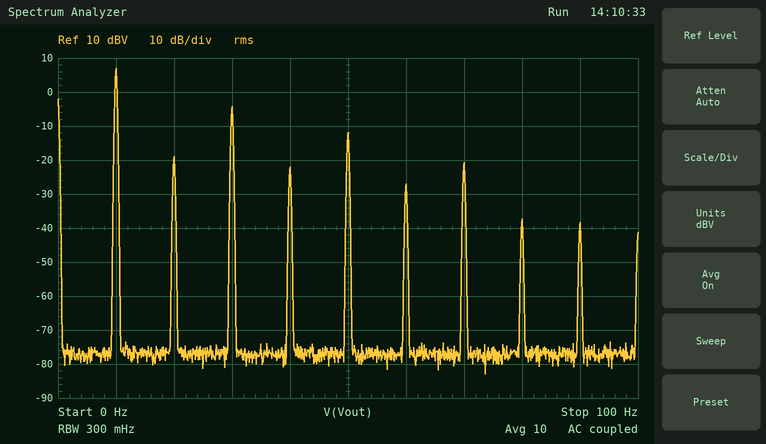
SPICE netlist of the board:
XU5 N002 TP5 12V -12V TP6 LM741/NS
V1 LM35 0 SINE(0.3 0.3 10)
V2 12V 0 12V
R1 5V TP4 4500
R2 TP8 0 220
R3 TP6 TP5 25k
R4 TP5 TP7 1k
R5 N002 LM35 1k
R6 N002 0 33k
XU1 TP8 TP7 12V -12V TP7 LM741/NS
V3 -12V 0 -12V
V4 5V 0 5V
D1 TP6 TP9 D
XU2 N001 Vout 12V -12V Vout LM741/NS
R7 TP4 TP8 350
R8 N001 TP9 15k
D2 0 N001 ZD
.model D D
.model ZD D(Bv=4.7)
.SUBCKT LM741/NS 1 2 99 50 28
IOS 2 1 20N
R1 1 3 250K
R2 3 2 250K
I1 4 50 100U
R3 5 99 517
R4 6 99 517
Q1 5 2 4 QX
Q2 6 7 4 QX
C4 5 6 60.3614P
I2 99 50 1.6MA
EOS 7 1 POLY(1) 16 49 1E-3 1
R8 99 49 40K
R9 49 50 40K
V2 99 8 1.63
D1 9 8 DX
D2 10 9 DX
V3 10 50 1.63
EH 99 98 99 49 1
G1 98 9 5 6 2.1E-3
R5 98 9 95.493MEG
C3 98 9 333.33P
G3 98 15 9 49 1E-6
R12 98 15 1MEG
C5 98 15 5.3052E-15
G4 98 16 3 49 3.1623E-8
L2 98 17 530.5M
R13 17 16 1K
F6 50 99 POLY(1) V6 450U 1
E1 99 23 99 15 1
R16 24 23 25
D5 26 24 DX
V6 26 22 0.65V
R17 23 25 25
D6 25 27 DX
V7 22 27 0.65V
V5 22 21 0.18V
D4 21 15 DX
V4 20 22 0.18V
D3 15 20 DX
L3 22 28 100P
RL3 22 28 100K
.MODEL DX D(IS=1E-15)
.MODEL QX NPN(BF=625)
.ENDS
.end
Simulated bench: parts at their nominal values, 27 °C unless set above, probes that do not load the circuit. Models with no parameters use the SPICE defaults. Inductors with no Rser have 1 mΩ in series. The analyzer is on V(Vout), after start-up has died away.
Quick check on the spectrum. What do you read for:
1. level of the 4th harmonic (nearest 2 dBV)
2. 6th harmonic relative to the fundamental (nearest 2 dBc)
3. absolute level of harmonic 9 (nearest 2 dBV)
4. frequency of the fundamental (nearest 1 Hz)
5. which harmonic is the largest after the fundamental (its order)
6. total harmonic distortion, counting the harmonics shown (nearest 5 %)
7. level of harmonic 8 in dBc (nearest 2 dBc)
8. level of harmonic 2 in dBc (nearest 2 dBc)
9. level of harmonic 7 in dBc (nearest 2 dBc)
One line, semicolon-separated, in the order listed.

-22 dBV; -34 dBc; -38 dBV; 10 Hz; 3; 30 %; -44 dBc; -26 dBc; -28 dBc
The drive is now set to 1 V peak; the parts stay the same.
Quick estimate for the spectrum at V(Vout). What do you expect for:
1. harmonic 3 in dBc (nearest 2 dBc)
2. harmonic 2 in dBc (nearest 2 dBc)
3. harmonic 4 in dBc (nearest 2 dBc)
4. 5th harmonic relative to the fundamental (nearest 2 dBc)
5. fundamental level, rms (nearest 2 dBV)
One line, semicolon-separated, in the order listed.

-10 dBc; -36 dBc; -36 dBc; -14 dBc; 8 dBV
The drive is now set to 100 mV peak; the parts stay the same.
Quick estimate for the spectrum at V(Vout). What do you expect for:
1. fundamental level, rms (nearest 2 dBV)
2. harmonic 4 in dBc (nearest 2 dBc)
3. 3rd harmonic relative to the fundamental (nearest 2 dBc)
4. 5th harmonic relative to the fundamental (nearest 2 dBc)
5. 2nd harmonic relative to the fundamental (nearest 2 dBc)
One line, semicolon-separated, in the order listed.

4 dBV; -34 dBc; -32 dBc; -36 dBc; -30 dBc
